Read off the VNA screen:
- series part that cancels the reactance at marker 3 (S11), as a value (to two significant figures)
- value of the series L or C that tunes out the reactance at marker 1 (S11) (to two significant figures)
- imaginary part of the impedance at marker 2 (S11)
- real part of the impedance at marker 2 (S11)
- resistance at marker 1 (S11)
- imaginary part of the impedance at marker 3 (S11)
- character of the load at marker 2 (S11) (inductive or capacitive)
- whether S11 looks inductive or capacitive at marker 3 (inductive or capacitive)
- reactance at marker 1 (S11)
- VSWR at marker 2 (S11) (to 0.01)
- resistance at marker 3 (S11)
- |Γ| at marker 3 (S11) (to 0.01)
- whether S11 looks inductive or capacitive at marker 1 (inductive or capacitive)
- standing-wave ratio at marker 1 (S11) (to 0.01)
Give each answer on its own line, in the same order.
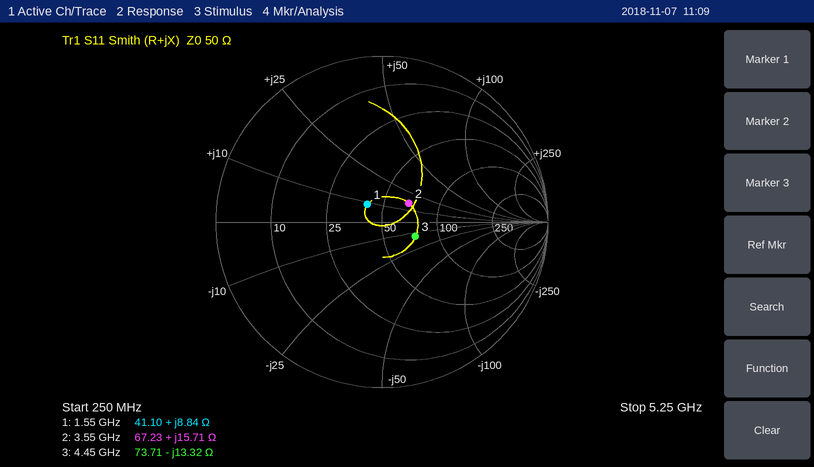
480 pH
12 pF
+15.71 Ω
67.23 Ω
41.10 Ω
-13.32 Ω
inductive
capacitive
+8.84 Ω
1.49
73.71 Ω
0.22
inductive
1.32
